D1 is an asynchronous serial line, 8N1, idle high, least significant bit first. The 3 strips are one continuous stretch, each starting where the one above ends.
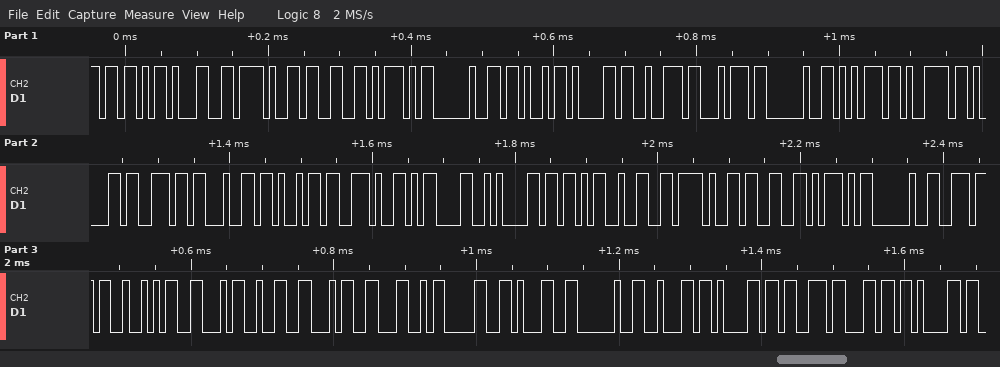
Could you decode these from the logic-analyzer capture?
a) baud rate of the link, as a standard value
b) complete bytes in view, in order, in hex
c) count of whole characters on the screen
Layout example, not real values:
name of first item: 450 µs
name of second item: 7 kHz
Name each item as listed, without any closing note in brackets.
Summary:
baud rate of the link, as a standard value: 115200 baud
complete bytes in view, in order, in hex: 0x5B 0x31 0x2F 0x33 0x5D 0x20 0x4B 0x61 0x72 0x74 0x20 0x75 0x79 0x61 0x6E 0x64 0x69 0x2E 0x0D 0x0A 0x5B 0x32 0x2F 0x33 0x5D 0x20 0x6E 0x52 0x46 0x32 0x34 0x4C 0x30 0x31 0x20 0x62 0x61 0x73 0x6C 0x61
count of whole characters on the screen: 40
